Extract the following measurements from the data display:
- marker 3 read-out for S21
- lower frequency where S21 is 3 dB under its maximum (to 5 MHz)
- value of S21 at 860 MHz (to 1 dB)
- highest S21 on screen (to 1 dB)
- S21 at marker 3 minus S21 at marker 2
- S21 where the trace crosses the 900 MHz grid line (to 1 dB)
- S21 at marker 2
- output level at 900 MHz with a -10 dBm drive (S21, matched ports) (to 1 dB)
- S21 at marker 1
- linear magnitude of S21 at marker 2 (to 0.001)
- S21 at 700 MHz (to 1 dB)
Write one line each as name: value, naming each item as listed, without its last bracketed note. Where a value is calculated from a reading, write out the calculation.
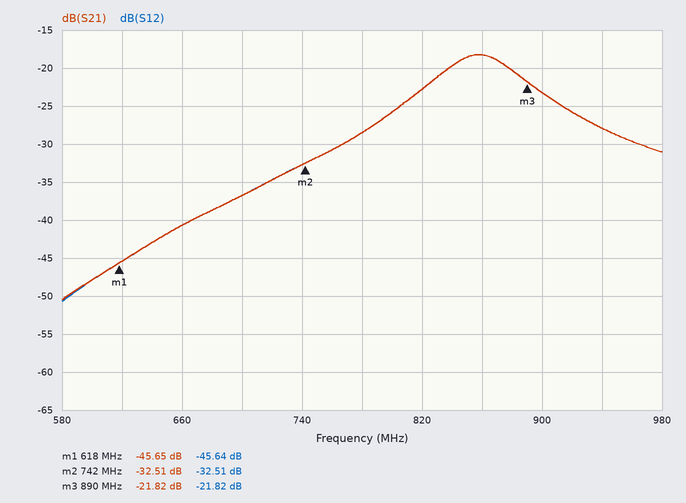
marker 3 read-out for S21: -21.82 dB
lower frequency where S21 is 3 dB under its maximum: 830 MHz
value of S21 at 860 MHz: -18 dB
highest S21 on screen: -18 dB
S21 at marker 3 minus S21 at marker 2: -21.82 − (-32.51) = 10.69 dB
S21 where the trace crosses the 900 MHz grid line: -23 dB
S21 at marker 2: -32.51 dB
output level at 900 MHz with a -10 dBm drive (S21, matched ports): -10 dBm + (-23 dB) = -33 dBm
S21 at marker 1: -45.65 dB
linear magnitude of S21 at marker 2: 10^(-32.51/20) ≈ 0.024
S21 at 700 MHz: -37 dB
